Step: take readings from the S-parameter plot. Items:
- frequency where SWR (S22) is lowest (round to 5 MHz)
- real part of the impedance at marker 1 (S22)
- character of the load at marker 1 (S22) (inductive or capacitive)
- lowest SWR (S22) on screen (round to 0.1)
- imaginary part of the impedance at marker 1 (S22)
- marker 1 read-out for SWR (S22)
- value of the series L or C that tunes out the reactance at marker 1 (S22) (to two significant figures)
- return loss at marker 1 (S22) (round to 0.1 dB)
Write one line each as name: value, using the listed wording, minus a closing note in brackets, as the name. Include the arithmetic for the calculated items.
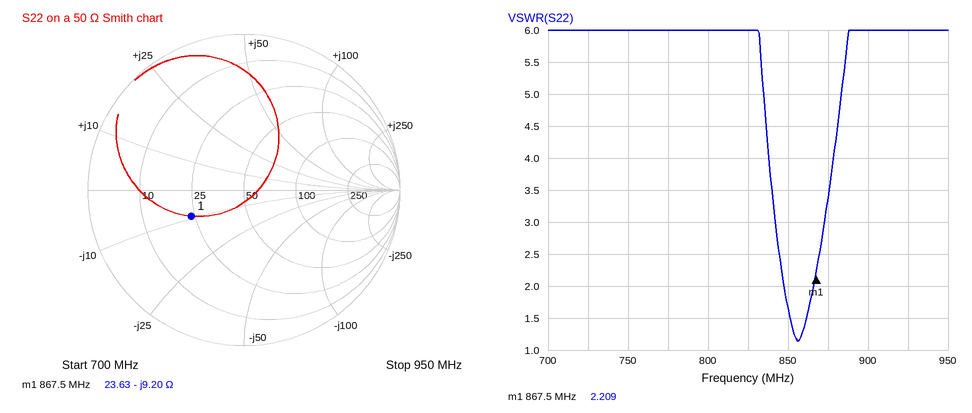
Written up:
frequency where SWR (S22) is lowest: 855 MHz
real part of the impedance at marker 1: 23.63 Ω
character of the load at marker 1 (S22): capacitive
lowest SWR (S22) on screen: 1.1
imaginary part of the impedance at marker 1: -9.20 Ω
marker 1 read-out for SWR: 2.209
value of the series L or C that tunes out the reactance at marker 1 (S22): L = 9.2 Ω/(2π × 867.5 MHz) ≈ 1.7 nH
return loss at marker 1 (S22): 8.5 dB
